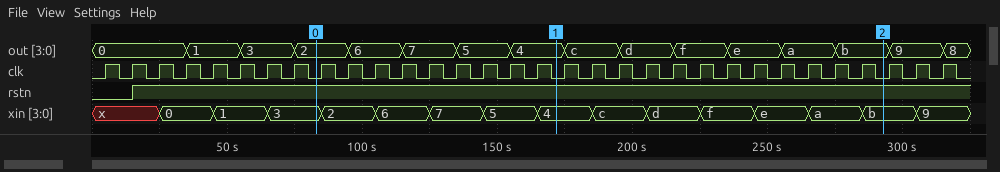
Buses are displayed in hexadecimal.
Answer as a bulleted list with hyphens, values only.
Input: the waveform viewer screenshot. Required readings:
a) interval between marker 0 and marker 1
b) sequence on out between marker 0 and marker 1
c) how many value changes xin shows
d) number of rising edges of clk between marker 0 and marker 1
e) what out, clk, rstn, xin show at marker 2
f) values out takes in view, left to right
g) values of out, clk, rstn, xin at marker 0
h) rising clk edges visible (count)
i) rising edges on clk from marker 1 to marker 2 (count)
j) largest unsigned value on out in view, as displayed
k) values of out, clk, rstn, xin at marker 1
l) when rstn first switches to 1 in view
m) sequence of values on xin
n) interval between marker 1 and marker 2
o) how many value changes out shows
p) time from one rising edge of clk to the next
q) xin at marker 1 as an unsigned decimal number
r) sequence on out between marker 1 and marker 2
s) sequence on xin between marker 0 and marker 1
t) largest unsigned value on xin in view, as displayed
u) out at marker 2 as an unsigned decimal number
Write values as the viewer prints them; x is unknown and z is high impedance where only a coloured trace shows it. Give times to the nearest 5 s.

- 90 s
- 2, 6, 7, 5, 4
- 15
- 9
- out=b, clk=0, rstn=1, xin=b
- 0, 1, 3, 2, 6, 7, 5, 4, c, d, f, e, a, b, 9, 8
- out=2, clk=0, rstn=1, xin=3
- 32
- 12
- f
- out=4, clk=0, rstn=1, xin=4
- 15 s
- x, 0, 1, 3, 2, 6, 7, 5, 4, c, d, f, e, a, b, 9
- 120 s
- 15
- 10 s
- 4
- 4, c, d, f, e, a, b
- 3, 2, 6, 7, 5, 4
- f
- 11
